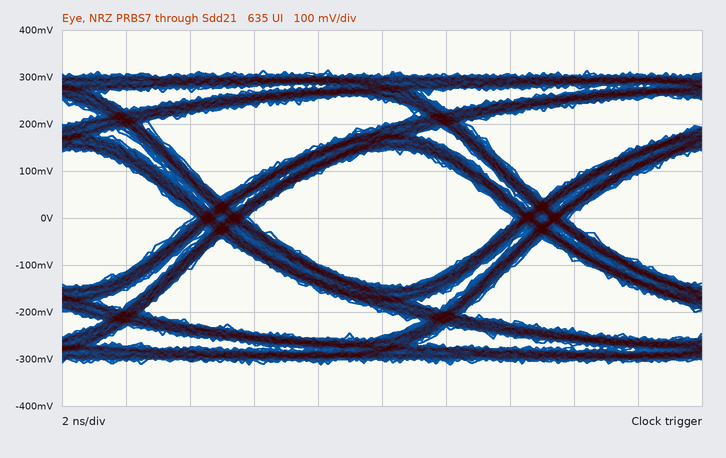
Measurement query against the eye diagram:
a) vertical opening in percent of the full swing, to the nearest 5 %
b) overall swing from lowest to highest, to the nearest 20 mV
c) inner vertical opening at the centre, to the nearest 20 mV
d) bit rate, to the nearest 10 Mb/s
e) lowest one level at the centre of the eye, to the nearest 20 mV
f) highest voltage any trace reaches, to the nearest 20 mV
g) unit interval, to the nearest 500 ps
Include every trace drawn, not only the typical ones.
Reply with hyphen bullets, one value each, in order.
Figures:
- 45 %
- 620 mV
- 280 mV
- 100 Mb/s
- 140 mV
- 320 mV
- 10.0 ns
